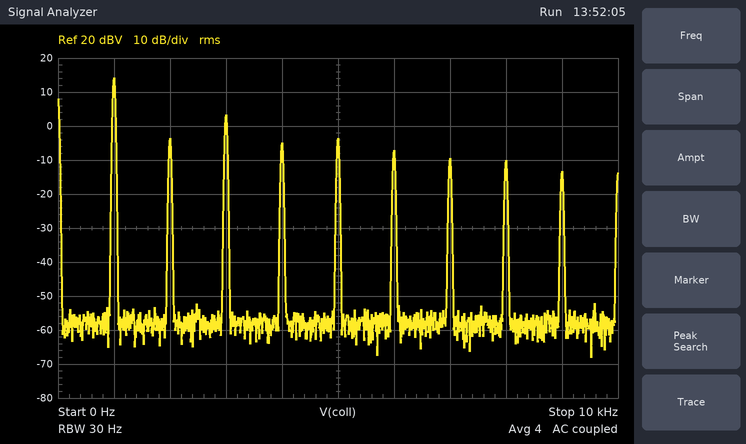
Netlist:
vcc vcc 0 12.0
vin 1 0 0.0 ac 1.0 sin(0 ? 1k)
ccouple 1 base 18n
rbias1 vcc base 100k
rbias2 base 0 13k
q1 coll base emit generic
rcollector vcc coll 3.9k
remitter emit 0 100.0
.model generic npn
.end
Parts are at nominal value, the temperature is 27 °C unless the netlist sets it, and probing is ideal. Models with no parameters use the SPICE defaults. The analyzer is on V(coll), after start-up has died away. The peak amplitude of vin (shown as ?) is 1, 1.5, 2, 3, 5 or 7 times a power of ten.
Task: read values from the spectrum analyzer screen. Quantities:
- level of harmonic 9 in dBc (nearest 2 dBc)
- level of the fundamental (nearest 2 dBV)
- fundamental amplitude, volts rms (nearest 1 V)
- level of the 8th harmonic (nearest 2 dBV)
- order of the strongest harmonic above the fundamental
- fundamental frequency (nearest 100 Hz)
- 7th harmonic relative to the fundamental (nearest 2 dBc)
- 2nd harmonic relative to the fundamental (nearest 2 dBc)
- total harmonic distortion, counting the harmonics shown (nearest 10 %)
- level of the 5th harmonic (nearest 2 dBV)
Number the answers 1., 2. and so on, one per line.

1. -28 dBc
2. 14 dBV
3. 5 V
4. -10 dBV
5. 3
6. 1.0 kHz
7. -24 dBc
8. -18 dBc
9. 40 %
10. -4 dBV
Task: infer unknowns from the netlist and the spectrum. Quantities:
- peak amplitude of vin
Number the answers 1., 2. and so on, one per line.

1. 2 V
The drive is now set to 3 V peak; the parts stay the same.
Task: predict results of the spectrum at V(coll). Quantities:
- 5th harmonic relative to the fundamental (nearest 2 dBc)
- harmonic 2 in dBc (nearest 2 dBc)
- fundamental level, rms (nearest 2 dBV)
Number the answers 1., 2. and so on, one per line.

1. -22 dBc
2. -14 dBc
3. 14 dBV
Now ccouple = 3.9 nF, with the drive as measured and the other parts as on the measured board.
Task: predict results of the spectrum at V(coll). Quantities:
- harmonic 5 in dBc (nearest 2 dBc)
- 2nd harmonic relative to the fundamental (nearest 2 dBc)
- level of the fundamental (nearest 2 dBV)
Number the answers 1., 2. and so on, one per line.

1. -34 dBc
2. -10 dBc
3. 12 dBV
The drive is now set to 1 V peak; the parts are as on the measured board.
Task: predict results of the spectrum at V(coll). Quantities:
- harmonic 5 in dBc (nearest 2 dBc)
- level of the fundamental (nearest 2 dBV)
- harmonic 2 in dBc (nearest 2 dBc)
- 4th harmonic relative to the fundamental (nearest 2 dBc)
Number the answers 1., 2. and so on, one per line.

1. -22 dBc
2. 14 dBV
3. -20 dBc
4. -22 dBc
